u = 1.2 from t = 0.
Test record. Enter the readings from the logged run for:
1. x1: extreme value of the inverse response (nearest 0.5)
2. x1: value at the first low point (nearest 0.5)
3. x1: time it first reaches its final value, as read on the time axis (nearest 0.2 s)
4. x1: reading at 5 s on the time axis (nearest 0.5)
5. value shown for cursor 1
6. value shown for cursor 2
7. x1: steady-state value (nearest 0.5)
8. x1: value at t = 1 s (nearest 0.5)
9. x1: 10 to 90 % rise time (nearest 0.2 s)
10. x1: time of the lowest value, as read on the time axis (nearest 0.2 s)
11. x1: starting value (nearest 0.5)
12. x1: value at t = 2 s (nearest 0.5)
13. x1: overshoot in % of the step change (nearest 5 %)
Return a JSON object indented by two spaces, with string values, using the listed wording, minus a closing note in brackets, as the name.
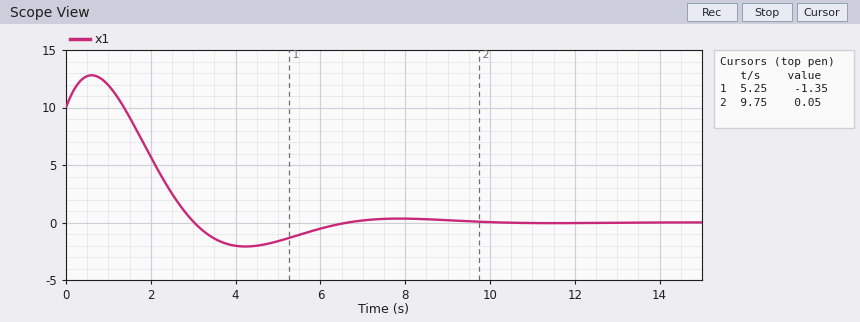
{
  "x1: extreme value of the inverse response": "13.0",
  "x1: value at the first low point": "-2.0",
  "x1: time it first reaches its final value, as read on the time axis": "3.0 s",
  "x1: reading at 5 s on the time axis": "-1.5",
  "value shown for cursor 1": "-1.35",
  "value shown for cursor 2": "0.05",
  "x1: steady-state value": "0.0",
  "x1: value at t = 1 s": "12.0",
  "x1: 10 to 90 % rise time": "1.2 s",
  "x1: time of the lowest value, as read on the time axis": "4.2 s",
  "x1: starting value": "10.0",
  "x1: value at t = 2 s": "5.5",
  "x1: overshoot in % of the step change": "20 %"
}
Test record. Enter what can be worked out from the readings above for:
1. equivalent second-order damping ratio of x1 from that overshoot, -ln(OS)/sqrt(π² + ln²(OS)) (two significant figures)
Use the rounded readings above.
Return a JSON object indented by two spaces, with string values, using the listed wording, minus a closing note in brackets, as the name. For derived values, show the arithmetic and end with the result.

{
  "equivalent second-order damping ratio of x1 from that overshoot, -ln(OS)/sqrt(π² + ln²(OS))": "ln(0.2) = -1.609; 1.609 / sqrt(9.870 + 2.590) = 0.46"
}
